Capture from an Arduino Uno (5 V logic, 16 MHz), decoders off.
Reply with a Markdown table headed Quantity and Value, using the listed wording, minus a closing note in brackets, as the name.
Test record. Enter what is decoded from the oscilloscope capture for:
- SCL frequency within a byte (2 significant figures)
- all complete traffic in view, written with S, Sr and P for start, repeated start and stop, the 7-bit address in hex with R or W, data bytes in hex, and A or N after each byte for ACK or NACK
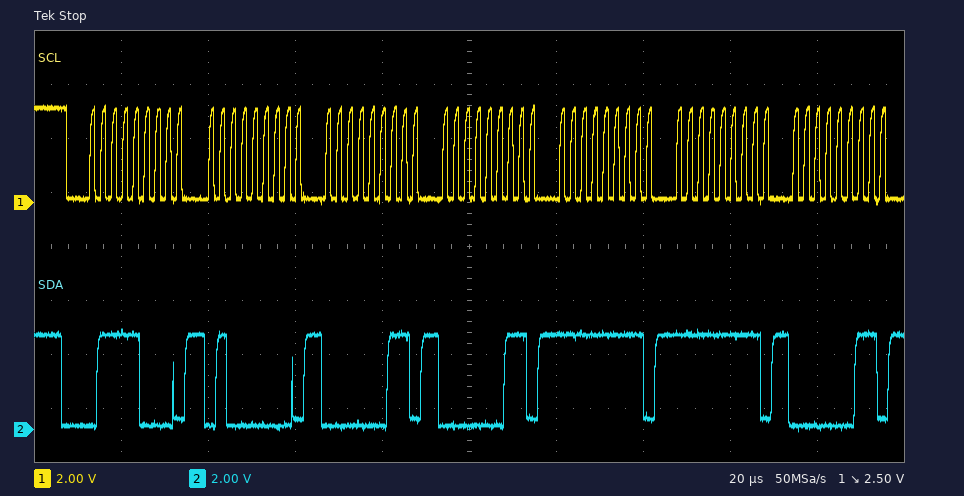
| Quantity | Value |
|---|---|
| SCL frequency within a byte | 400 kHz |
| all complete traffic in view, written with S, Sr and P for start, repeated start and stop, the 7-bit address in hex with R or W, data bytes in hex, and A or N after each byte for ACK or NACK | S 3CW A 40 A 03 A 03 A FF A FF A 03 A |
